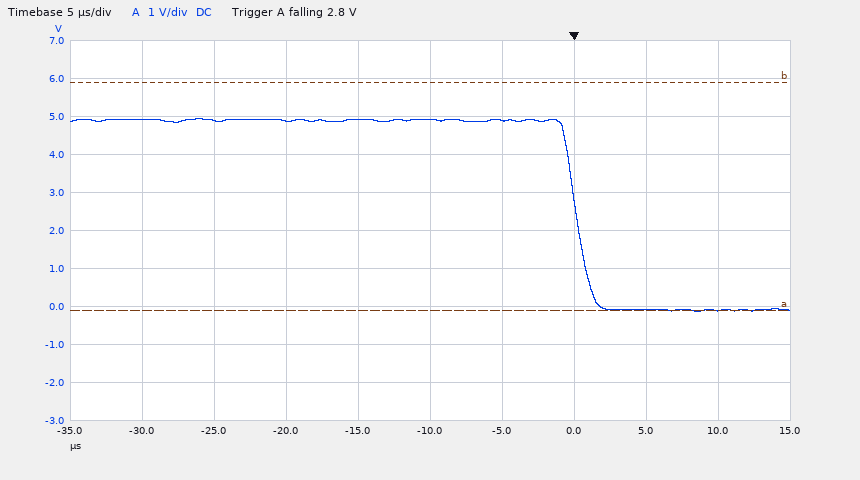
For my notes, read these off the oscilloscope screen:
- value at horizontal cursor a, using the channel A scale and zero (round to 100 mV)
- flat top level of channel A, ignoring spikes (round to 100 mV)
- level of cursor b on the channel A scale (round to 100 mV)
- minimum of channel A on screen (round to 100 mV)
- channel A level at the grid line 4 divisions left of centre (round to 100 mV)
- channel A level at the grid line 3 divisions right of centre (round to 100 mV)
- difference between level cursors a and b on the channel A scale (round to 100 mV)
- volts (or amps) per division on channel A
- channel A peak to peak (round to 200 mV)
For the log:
-100 mV
4.9 V
5.9 V
-100 mV
4.9 V
-100 mV
6.0 V
1 V
5.0 V
